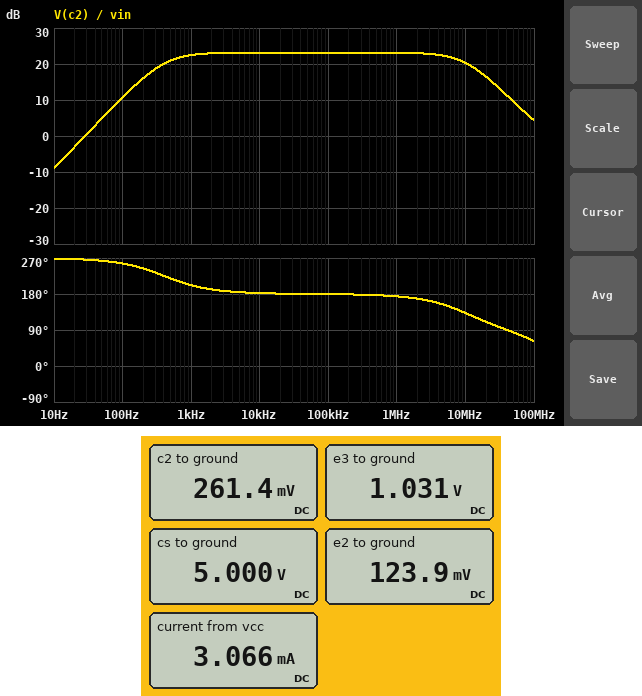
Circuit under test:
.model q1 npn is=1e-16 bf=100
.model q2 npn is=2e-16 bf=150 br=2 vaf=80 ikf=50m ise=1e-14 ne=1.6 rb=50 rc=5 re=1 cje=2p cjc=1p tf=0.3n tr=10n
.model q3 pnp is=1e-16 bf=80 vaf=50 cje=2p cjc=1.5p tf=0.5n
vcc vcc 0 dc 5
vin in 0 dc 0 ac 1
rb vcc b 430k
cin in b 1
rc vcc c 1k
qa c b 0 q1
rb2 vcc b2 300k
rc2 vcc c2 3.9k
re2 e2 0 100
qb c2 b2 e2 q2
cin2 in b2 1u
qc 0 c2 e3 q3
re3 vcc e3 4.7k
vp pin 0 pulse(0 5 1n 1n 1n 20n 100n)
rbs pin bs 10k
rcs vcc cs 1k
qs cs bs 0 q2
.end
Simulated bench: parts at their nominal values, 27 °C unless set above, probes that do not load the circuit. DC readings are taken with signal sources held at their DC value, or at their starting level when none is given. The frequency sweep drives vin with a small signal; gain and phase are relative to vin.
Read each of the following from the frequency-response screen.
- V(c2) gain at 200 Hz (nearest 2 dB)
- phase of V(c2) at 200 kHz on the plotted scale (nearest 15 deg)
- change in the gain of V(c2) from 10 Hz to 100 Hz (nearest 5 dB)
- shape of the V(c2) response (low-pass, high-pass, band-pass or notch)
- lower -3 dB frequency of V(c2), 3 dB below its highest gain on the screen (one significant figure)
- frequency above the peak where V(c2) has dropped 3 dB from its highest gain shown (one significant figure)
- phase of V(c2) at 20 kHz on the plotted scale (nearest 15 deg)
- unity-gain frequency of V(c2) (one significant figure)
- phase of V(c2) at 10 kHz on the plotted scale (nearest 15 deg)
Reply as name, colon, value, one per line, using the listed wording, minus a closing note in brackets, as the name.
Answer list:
V(c2) gain at 200 Hz: 16 dB
phase of V(c2) at 200 kHz on the plotted scale: 180 deg
change in the gain of V(c2) from 10 Hz to 100 Hz: 20 dB
shape of the V(c2) response: band-pass
lower -3 dB frequency of V(c2), 3 dB below its highest gain on the screen: 400 Hz
frequency above the peak where V(c2) has dropped 3 dB from its highest gain shown: 10 MHz
phase of V(c2) at 20 kHz on the plotted scale: 180 deg
unity-gain frequency of V(c2): 30 Hz
phase of V(c2) at 10 kHz on the plotted scale: 180 deg
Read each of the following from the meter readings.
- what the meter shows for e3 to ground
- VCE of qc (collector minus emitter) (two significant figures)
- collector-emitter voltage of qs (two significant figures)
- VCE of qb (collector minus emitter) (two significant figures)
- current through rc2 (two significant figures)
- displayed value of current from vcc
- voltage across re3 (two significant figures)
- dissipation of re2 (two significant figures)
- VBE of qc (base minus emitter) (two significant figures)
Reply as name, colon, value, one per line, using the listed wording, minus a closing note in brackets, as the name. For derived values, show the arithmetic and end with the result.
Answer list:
what the meter shows for e3 to ground: 1.031 V
VCE of qc (collector minus emitter): 0 V - 1.031 V = -1.0 V
collector-emitter voltage of qs: 5 V = 5.0 V
VCE of qb (collector minus emitter): 261.4 mV - 123.9 mV = 140 mV
current through rc2: (5 V - 261.4 mV) / 3.9 kΩ = 1.2 mA
displayed value of current from vcc: 3.066 mA
voltage across re3: 5 V - 1.031 V = 4.0 V
dissipation of re2: (123.9 mV)^2 / 100 Ω = 150 µW
VBE of qc (base minus emitter): 261.4 mV - 1.031 V = -770 mV
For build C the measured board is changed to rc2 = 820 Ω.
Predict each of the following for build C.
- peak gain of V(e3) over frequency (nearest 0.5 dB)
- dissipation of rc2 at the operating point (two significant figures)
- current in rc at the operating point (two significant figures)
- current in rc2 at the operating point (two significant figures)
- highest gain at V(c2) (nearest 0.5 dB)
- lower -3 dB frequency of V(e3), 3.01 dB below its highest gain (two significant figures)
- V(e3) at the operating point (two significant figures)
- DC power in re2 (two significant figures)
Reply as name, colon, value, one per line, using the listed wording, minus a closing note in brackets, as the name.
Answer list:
peak gain of V(e3) over frequency: 16.5 dB
dissipation of rc2 at the operating point: 2.7 mW
current in rc at the operating point: 980 µA
current in rc2 at the operating point: 1.8 mA
highest gain at V(c2): 17.0 dB
lower -3 dB frequency of V(e3), 3.01 dB below its highest gain: 11 Hz
V(e3) at the operating point: 4.2 V
DC power in re2: 340 µW
